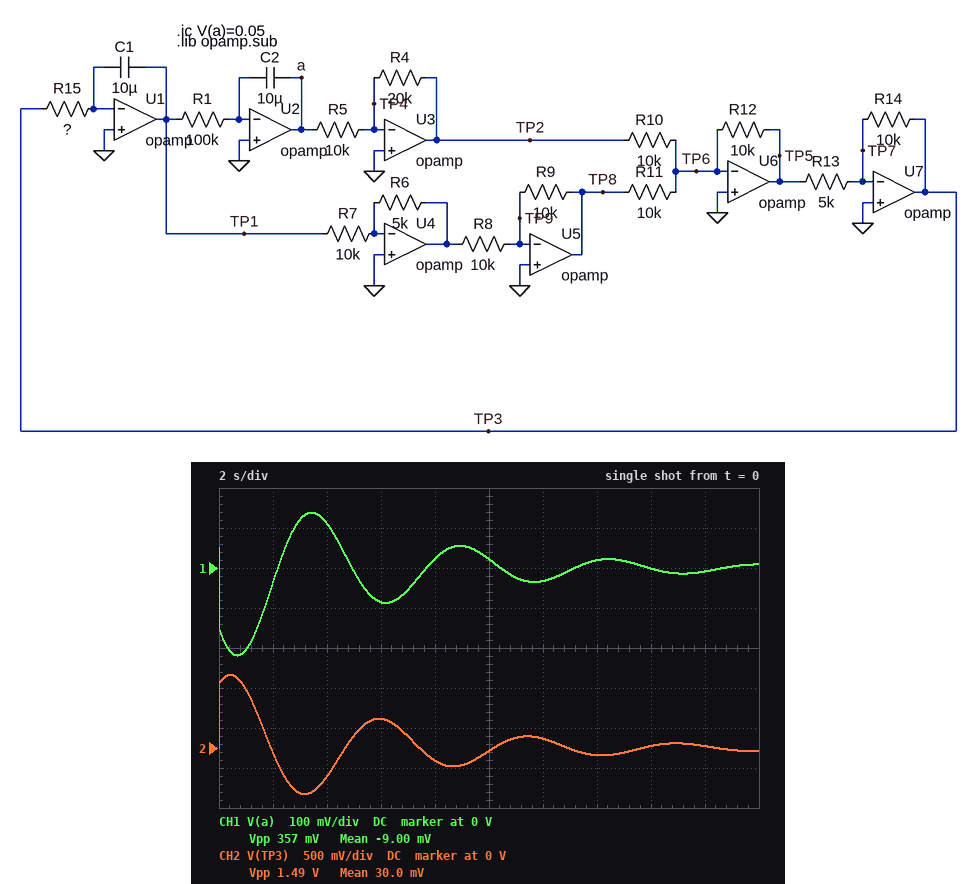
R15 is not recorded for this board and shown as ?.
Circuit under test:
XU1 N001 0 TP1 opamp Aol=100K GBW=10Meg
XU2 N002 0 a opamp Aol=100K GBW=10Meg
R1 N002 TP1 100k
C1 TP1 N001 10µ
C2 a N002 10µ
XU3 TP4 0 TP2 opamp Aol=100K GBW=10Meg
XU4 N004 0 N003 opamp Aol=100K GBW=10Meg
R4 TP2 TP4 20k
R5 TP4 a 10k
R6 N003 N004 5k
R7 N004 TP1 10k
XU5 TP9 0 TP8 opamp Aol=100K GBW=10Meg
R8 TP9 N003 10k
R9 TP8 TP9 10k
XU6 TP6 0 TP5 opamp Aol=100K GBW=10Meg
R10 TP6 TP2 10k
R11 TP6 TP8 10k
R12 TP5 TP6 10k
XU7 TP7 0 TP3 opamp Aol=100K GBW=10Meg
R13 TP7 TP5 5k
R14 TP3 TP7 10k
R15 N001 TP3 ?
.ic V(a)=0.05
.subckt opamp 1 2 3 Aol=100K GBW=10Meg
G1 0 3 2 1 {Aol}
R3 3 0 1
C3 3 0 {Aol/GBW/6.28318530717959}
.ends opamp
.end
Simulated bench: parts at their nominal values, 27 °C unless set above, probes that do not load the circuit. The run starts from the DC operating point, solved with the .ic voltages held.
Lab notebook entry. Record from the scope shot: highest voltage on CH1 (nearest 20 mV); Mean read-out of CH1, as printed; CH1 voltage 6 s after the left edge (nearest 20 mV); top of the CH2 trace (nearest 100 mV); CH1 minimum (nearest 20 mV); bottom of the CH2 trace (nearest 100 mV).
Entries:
140 mV
-9.00 mV
-80 mV
900 mV
-220 mV
-600 mV
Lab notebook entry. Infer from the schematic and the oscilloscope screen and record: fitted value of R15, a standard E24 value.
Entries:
300 kΩ
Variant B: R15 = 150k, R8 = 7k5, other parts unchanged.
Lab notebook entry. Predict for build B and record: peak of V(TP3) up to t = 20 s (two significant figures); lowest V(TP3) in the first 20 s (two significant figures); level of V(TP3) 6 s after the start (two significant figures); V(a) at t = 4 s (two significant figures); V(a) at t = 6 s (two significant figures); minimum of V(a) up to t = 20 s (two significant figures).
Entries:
600 mV
-250 mV
-42 mV
-17 mV
7.0 mV
-130 mV
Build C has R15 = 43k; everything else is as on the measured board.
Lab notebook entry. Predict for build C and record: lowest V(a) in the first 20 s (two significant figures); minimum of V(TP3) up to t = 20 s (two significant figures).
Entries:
-160 mV
-240 mV
